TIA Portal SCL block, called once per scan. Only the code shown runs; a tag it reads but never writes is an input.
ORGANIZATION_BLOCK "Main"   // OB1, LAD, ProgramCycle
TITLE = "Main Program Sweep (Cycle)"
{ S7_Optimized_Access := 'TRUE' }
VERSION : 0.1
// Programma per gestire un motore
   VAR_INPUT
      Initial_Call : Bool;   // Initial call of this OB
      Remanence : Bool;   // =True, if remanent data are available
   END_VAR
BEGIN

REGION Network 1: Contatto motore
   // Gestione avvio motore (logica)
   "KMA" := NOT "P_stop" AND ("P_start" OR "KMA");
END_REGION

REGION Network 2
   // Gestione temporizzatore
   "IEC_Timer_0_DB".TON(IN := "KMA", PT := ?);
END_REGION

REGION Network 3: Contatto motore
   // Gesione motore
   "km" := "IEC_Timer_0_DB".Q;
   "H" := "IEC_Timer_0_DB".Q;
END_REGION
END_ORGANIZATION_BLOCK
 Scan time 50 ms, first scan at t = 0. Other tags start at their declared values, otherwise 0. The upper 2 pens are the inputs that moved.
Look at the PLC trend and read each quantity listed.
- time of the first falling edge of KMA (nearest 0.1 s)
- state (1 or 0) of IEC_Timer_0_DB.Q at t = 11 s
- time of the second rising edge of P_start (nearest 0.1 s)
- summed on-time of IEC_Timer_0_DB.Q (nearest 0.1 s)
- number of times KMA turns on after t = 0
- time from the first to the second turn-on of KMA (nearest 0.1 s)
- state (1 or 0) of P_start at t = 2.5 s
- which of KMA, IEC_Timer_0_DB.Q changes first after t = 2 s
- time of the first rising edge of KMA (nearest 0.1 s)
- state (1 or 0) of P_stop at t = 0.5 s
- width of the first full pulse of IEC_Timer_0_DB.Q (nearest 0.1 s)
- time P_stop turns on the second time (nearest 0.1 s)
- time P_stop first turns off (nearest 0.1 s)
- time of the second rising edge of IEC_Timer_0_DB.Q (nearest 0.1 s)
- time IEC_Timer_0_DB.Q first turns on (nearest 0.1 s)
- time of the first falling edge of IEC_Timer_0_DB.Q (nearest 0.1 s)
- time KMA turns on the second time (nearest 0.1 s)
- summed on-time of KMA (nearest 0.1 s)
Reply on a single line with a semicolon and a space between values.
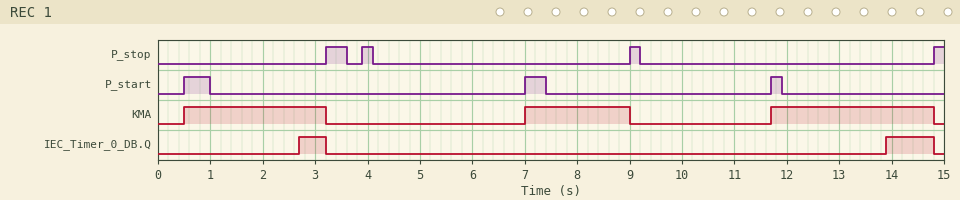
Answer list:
3.2 s; 0; 7.0 s; 1.4 s; 3; 6.5 s; 0; IEC_Timer_0_DB.Q; 0.5 s; 0; 0.5 s; 3.9 s; 3.6 s; 13.9 s; 2.7 s; 3.2 s; 7.0 s; 7.8 s
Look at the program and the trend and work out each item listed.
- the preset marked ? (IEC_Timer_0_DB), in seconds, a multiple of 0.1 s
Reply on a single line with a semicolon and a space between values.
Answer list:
2.2 s
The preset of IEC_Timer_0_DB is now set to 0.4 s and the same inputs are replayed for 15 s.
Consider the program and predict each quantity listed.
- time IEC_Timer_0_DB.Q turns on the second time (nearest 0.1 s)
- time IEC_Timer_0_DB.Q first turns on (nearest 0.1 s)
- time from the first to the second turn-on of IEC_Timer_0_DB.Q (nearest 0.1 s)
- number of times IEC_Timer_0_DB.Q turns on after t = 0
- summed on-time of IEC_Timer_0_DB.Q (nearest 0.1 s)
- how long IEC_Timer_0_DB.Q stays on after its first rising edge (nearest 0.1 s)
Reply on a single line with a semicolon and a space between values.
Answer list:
7.4 s; 0.9 s; 6.5 s; 3; 6.6 s; 2.3 s
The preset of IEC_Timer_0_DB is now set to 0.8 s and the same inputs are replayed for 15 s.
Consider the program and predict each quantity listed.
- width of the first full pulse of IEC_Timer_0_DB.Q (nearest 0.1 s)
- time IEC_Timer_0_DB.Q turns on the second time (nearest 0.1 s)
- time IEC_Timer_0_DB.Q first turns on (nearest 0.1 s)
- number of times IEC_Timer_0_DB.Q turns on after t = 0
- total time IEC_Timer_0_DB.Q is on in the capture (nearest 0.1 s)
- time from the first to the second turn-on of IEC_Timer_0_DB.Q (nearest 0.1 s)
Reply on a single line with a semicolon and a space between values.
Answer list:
1.9 s; 7.8 s; 1.3 s; 3; 5.4 s; 6.5 s
